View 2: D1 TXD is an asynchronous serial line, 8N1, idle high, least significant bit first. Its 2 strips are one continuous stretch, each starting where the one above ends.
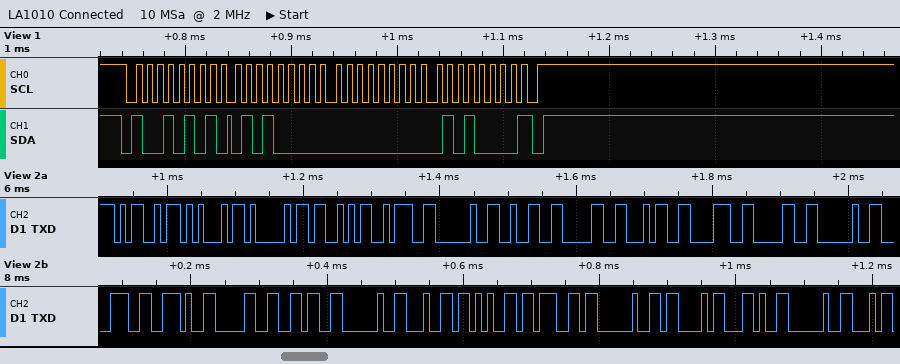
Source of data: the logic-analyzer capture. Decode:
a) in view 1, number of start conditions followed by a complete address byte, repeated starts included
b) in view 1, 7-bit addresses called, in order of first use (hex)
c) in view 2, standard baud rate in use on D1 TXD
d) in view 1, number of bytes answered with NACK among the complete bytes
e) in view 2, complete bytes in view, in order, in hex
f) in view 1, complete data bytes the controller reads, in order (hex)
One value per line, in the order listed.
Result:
1
0x4A
115200 baud
1
4D 45 41 53 3A 20 32 30 34 38 30 20 38 2E 30 36 20 64 65 67 20 43 2C 20
50 00 50
